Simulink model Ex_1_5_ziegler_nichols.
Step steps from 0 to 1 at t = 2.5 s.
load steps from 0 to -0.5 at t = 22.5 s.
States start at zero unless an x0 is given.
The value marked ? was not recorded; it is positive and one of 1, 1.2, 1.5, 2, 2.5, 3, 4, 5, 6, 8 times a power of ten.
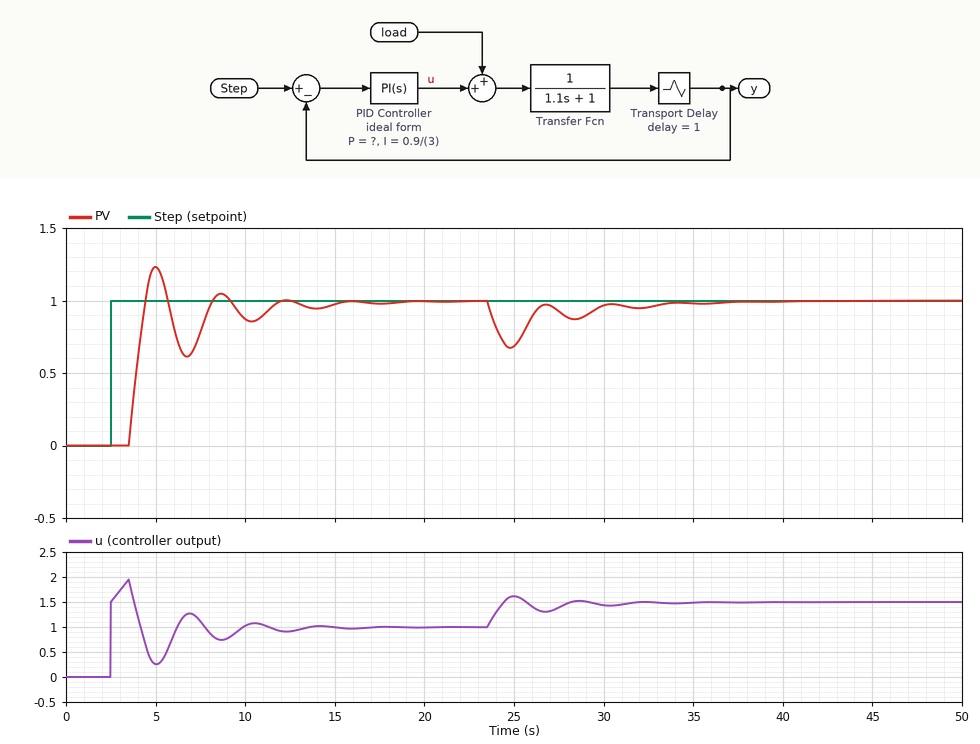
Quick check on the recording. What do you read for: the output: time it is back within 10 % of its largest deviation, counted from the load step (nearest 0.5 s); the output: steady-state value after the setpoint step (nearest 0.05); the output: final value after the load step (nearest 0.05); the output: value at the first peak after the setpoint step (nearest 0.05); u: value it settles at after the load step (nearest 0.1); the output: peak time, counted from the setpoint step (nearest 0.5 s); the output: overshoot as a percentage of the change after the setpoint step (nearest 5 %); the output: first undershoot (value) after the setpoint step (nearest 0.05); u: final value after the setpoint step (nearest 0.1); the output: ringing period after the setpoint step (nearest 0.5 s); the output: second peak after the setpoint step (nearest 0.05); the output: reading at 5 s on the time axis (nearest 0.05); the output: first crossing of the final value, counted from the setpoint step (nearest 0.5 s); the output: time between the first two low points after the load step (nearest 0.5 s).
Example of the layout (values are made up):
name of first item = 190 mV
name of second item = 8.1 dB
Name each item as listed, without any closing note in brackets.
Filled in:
the output: time it is back within 10 % of its largest deviation, counted from the load step = 10.5 s
the output: steady-state value after the setpoint step = 1.00
the output: final value after the load step = 1.00
the output: value at the first peak after the setpoint step = 1.25
u: value it settles at after the load step = 1.5
the output: peak time, counted from the setpoint step = 2.5 s
the output: overshoot as a percentage of the change after the setpoint step = 25 %
the output: first undershoot (value) after the setpoint step = 0.60
u: final value after the setpoint step = 1.0
the output: ringing period after the setpoint step = 3.5 s
the output: second peak after the setpoint step = 1.05
the output: reading at 5 s on the time axis = 1.25
the output: first crossing of the final value, counted from the setpoint step = 2.0 s
the output: time between the first two low points after the load step = 3.5 s
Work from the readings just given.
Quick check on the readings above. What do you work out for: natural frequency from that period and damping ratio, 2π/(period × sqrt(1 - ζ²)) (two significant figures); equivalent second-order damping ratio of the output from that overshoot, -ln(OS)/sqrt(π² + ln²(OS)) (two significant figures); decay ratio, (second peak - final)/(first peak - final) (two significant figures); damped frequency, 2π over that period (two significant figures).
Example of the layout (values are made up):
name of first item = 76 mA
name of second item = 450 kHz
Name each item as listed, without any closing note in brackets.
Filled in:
natural frequency from that period and damping ratio, 2π/(period × sqrt(1 - ζ²)) = 2.0 rad/s
equivalent second-order damping ratio of the output from that overshoot, -ln(OS)/sqrt(π² + ln²(OS)) = 0.40
decay ratio, (second peak - final)/(first peak - final) = 0.20
damped frequency, 2π over that period = 1.8 rad/s
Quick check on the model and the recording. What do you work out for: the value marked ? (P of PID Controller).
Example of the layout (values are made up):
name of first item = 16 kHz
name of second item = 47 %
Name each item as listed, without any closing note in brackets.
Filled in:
the value marked ? = 1.5
